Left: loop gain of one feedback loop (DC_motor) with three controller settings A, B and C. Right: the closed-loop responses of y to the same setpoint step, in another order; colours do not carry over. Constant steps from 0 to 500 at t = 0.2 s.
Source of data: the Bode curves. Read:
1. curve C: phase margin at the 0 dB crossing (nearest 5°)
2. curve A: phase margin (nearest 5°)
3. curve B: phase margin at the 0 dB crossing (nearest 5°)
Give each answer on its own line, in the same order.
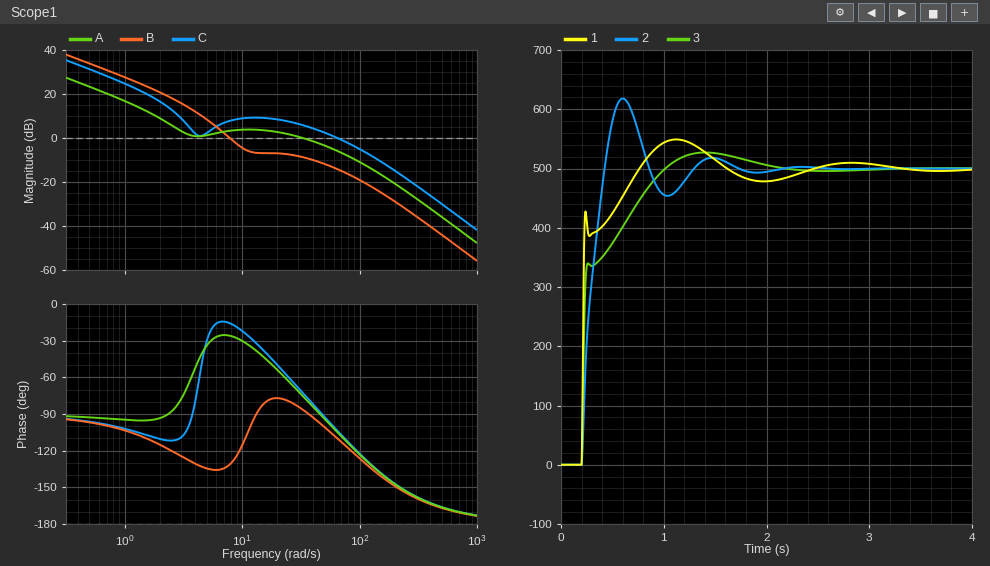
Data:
75°
105°
50°
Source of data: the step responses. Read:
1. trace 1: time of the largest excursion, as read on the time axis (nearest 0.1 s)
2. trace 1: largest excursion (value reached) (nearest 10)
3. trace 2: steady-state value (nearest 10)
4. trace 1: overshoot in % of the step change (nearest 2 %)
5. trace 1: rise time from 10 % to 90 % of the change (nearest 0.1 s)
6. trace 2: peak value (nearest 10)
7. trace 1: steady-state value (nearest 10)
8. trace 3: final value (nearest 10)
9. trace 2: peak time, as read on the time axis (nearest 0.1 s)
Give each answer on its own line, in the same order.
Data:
1.1 s
550
500
10 %
0.4 s
620
500
500
0.6 s
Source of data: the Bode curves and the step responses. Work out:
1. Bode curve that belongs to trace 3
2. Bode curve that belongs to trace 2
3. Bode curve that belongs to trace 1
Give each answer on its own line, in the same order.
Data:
A
B
C
